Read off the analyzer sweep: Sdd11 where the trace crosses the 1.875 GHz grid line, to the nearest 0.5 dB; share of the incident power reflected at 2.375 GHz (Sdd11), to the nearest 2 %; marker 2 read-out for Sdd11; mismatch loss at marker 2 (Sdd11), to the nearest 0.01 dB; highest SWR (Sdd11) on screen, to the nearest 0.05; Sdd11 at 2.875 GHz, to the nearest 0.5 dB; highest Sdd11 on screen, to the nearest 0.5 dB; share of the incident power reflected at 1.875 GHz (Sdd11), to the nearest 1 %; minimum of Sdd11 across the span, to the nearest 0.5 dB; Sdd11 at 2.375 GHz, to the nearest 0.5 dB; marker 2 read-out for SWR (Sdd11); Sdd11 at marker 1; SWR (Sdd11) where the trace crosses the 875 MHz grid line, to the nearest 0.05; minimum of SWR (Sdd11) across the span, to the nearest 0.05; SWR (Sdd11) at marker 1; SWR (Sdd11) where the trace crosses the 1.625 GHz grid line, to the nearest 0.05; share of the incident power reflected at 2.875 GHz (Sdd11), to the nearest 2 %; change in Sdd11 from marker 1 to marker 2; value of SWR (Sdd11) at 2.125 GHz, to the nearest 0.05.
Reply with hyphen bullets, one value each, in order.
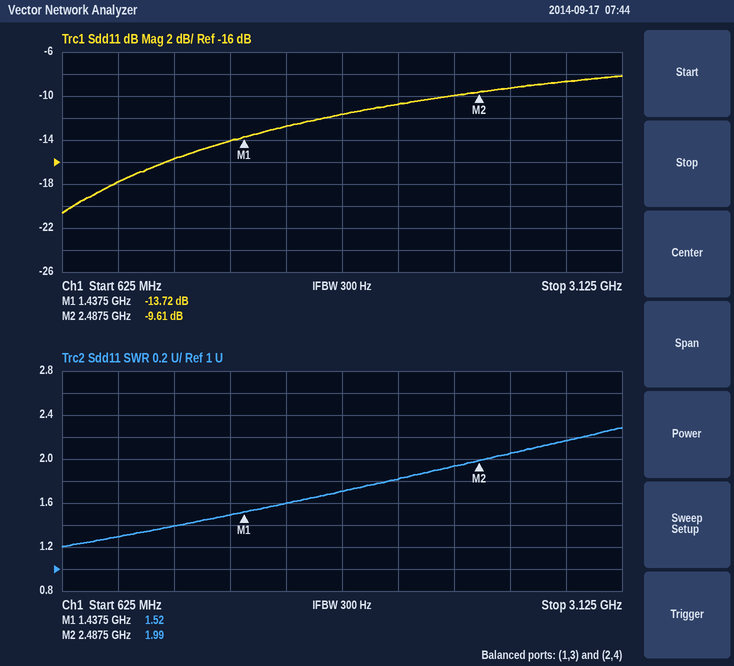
- -11.5 dB
- 10 %
- -9.61 dB
- 0.50 dB
- 2.30
- -8.5 dB
- -8.0 dB
- 7 %
- -20.5 dB
- -10.0 dB
- 1.99
- -13.72 dB
- 1.30
- 1.20
- 1.52
- 1.60
- 14 %
- 4.11 dB
- 1.80
